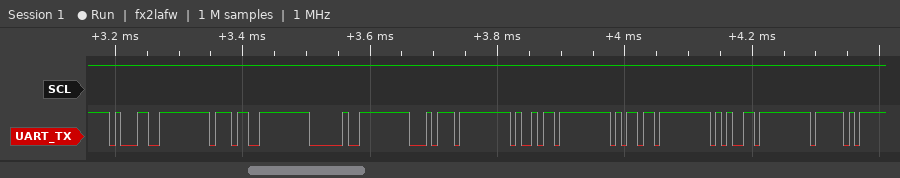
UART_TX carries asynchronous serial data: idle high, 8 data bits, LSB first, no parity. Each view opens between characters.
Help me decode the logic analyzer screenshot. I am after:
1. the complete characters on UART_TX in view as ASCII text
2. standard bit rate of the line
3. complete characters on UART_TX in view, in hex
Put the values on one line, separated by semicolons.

"17 time_"; 115200 baud; 31, 37, 20, 74, 69, 6D, 65, 5F
